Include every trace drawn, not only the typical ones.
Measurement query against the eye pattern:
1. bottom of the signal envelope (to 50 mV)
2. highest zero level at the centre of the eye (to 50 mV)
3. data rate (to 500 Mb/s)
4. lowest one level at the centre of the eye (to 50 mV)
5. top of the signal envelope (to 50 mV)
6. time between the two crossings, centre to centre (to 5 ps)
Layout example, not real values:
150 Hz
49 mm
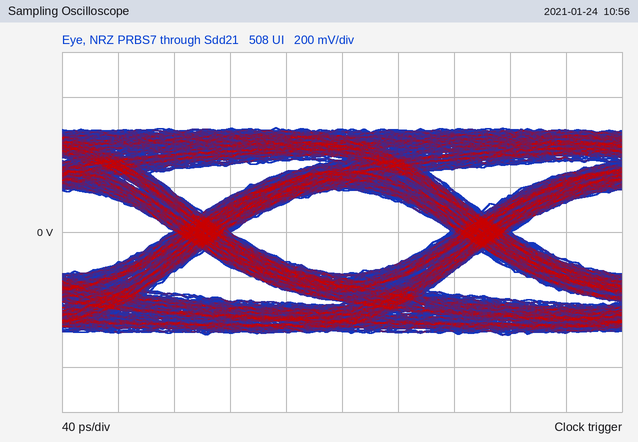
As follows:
-450 mV
-200 mV
5.0 Gb/s
200 mV
450 mV
200 ps
